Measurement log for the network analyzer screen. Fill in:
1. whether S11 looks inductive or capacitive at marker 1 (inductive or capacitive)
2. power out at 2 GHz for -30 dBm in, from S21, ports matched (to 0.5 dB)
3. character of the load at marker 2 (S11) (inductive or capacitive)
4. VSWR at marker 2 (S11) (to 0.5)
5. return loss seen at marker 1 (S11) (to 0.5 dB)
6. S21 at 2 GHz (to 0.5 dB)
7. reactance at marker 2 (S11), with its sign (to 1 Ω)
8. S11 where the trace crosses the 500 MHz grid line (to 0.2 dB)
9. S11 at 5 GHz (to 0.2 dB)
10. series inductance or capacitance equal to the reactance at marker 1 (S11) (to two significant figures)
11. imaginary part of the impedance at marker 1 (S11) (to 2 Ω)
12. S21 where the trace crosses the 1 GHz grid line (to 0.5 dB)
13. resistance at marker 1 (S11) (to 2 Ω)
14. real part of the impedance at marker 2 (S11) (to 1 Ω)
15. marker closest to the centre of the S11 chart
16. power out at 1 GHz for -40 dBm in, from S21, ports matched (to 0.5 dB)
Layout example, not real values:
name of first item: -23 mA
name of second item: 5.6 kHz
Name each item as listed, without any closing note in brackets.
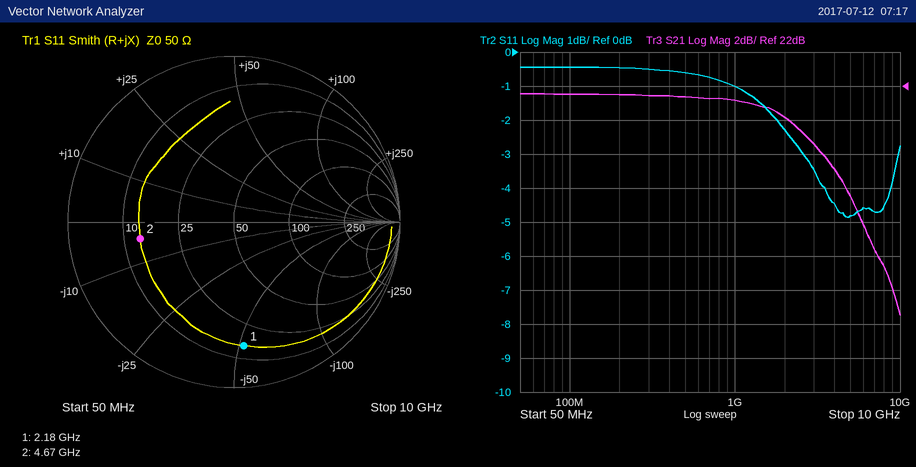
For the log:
whether S11 looks inductive or capacitive at marker 1: capacitive
power out at 2 GHz for -30 dBm in, from S21, ports matched: -10.0 dBm
character of the load at marker 2 (S11): capacitive
VSWR at marker 2 (S11): 3.5
return loss seen at marker 1 (S11): 2.5 dB
S21 at 2 GHz: 20.0 dB
reactance at marker 2 (S11), with its sign: -4 Ω
S11 where the trace crosses the 500 MHz grid line: -0.6 dB
S11 at 5 GHz: -4.8 dB
series inductance or capacitance equal to the reactance at marker 1 (S11): 1.4 pF
imaginary part of the impedance at marker 1 (S11): -52 Ω
S21 where the trace crosses the 1 GHz grid line: 21.0 dB
resistance at marker 1 (S11): 16 Ω
real part of the impedance at marker 2 (S11): 14 Ω
marker closest to the centre of the S11 chart: marker 2
power out at 1 GHz for -40 dBm in, from S21, ports matched: -19.0 dBm
